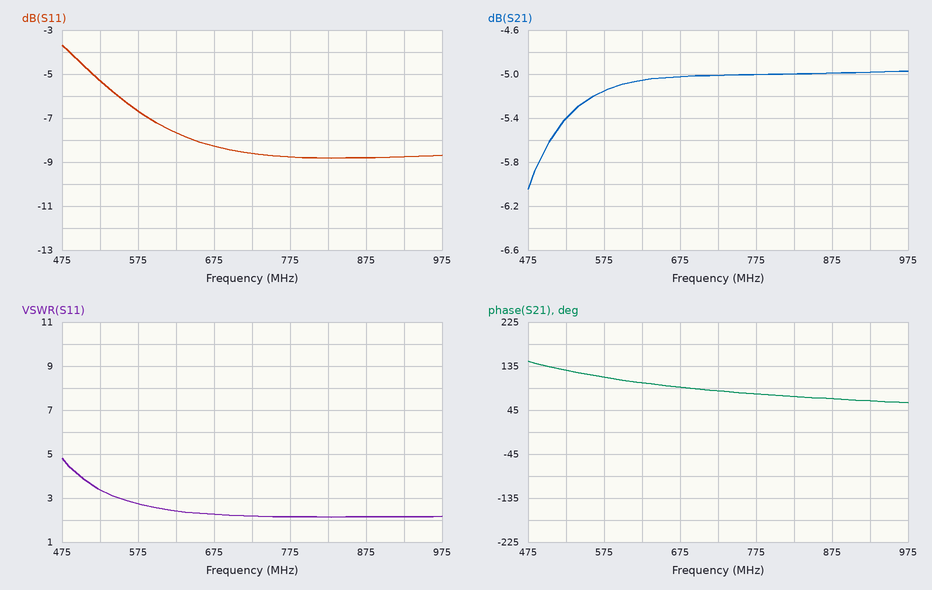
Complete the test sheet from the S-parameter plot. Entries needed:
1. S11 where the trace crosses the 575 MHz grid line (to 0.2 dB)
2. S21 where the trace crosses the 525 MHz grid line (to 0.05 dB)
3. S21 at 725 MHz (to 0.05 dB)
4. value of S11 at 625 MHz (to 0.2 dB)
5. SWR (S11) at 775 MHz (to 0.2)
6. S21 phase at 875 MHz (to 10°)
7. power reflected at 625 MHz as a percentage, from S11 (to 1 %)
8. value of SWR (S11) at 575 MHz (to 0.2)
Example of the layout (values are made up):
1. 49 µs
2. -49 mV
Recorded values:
1. -6.6 dB
2. -5.40 dB
3. -5.00 dB
4. -7.6 dB
5. 2.2
6. 70°
7. 17 %
8. 2.8
